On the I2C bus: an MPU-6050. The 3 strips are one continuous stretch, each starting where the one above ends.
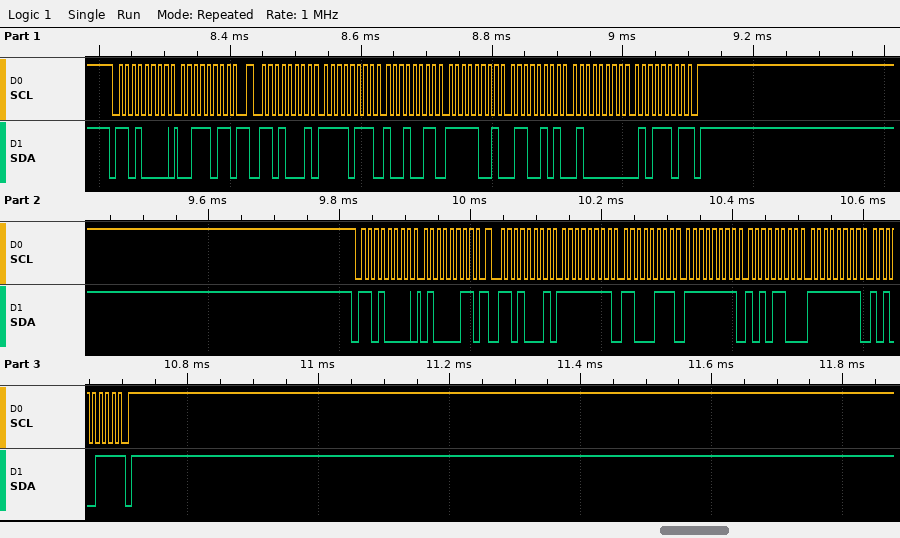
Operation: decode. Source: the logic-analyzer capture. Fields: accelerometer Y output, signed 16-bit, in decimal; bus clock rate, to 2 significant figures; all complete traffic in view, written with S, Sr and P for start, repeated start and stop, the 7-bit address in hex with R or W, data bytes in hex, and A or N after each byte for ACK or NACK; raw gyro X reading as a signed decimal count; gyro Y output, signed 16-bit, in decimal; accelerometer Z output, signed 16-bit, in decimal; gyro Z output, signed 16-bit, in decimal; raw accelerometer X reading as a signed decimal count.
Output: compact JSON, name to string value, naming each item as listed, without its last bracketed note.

{"accelerometer Y output, signed 16-bit, in decimal": "-1691", "bus clock rate, to 2 significant figures": "100 kHz", "all complete traffic in view, written with S, Sr and P for start, repeated start and stop, the 7-bit address in hex with R or W, data bytes in hex, and A or N after each byte for ACK or NACK": "S 68W A 3B A Sr 68R A F7 A 93 A F9 A 65 A 40 A 5D N P S 68W A 43 A Sr 68R A FF A C7 A FF A AC A FF A A7 N P", "raw gyro X reading as a signed decimal count": "-57", "gyro Y output, signed 16-bit, in decimal": "-84", "accelerometer Z output, signed 16-bit, in decimal": "16477", "gyro Z output, signed 16-bit, in decimal": "-89", "raw accelerometer X reading as a signed decimal count": "-2157"}
